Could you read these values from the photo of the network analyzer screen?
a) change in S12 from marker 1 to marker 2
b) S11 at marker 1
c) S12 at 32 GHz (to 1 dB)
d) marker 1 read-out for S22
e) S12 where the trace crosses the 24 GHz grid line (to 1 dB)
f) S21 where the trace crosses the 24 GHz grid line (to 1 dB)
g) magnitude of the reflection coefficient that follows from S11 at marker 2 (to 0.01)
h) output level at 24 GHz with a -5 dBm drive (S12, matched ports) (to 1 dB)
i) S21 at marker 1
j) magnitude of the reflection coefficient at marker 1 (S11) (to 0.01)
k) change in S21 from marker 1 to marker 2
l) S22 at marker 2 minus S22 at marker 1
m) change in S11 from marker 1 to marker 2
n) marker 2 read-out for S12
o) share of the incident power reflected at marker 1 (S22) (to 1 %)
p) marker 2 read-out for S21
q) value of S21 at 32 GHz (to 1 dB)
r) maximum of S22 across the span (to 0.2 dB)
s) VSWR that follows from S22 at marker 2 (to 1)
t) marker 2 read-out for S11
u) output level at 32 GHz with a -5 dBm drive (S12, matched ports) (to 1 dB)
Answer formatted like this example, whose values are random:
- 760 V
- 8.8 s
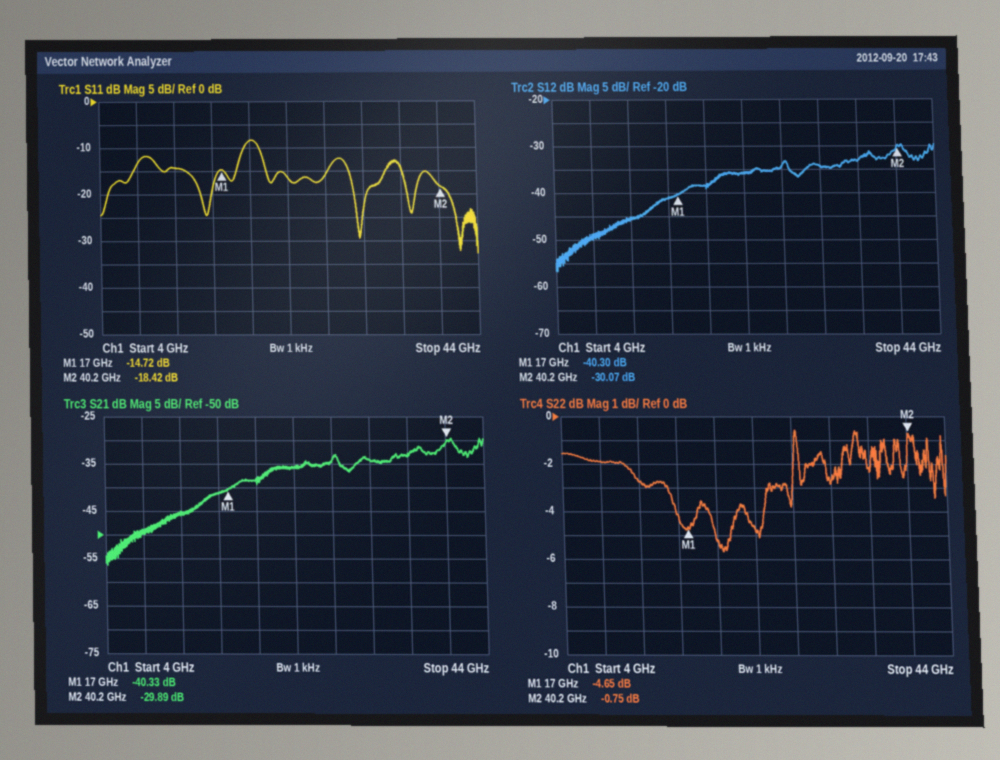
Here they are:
- 10.23 dB
- -14.72 dB
- -34 dB
- -4.65 dB
- -36 dB
- -36 dB
- 0.12
- -41 dBm
- -40.33 dB
- 0.18
- 10.44 dB
- 3.90 dB
- -3.70 dB
- -30.07 dB
- 34 %
- -29.89 dB
- -34 dB
- -0.6 dB
- 23
- -18.42 dB
- -39 dBm
